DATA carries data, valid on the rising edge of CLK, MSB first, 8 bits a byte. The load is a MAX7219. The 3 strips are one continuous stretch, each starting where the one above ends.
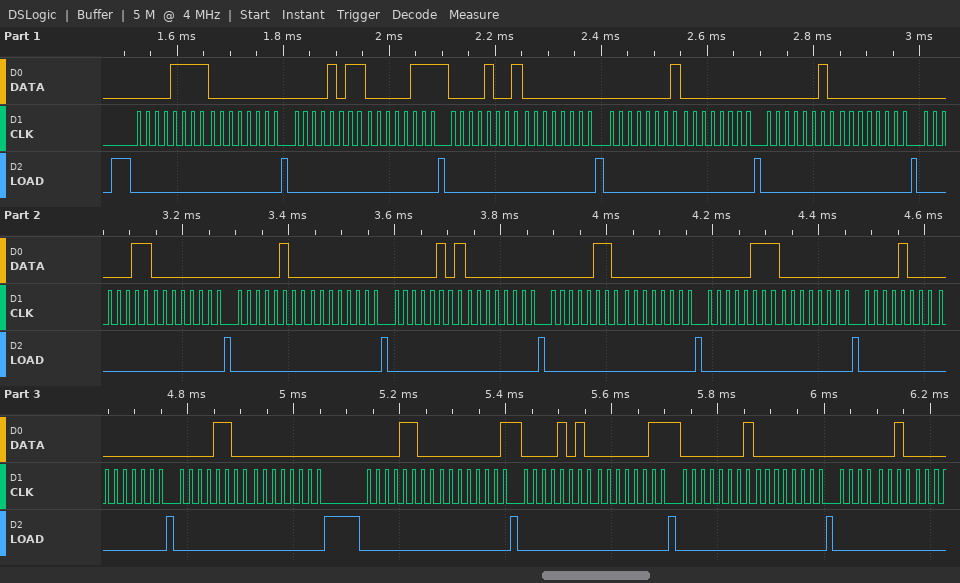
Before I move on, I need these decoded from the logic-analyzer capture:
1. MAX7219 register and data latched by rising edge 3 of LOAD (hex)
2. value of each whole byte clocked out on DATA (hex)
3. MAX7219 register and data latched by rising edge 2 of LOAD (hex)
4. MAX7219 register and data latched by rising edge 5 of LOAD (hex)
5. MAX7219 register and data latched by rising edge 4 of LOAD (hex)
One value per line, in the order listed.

register 0xB, data 0x07
0F 00 0B 07 09 00 01 00 02 00 03 00 04 00 05 00 06 00 07 00 08 00 0C 00 0C 01 0A 03 01 00 02
register 0xF, data 0x00
register 0x1, data 0x00
register 0x9, data 0x00
